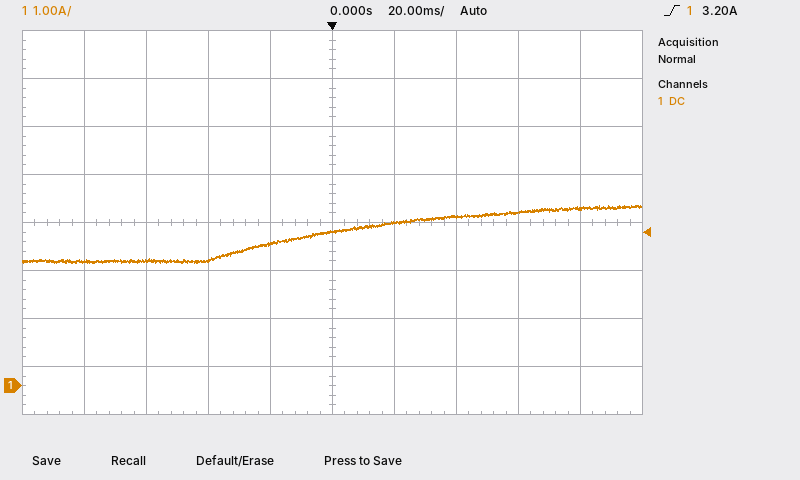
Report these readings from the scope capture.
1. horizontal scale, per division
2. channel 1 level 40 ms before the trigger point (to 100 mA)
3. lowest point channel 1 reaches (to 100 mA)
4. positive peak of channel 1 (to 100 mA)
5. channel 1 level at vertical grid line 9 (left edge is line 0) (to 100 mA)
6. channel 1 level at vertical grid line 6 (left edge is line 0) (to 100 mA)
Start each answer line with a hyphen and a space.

- 20 ms
- 2.6 A
- 2.5 A
- 3.8 A
- 3.7 A
- 3.4 A
